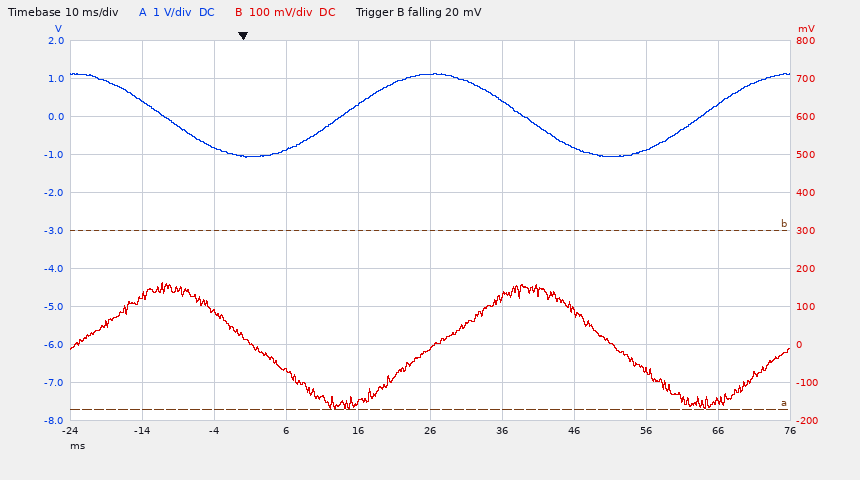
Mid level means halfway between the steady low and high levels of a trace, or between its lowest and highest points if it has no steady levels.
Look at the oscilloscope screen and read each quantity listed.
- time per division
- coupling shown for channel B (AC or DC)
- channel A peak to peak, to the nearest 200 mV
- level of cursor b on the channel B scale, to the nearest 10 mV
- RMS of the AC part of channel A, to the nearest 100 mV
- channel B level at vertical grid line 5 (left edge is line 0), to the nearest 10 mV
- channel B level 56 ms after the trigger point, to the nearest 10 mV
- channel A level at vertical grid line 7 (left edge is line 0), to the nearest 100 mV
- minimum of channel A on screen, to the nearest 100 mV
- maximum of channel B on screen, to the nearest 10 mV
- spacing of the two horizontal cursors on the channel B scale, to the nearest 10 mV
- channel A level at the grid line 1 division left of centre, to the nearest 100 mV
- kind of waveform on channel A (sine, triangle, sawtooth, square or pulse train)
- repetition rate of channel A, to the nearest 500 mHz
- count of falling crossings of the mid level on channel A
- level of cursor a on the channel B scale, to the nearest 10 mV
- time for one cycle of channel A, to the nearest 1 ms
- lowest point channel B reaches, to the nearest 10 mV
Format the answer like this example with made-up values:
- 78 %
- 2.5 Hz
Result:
- 10 ms
- DC
- 2.2 V
- 300 mV
- 800 mV
- -10 mV
- -70 mV
- -800 mV
- -1.1 V
- 160 mV
- 470 mV
- 300 mV
- sine
- 20.0 Hz
- 2
- -170 mV
- 50 ms
- -170 mV
